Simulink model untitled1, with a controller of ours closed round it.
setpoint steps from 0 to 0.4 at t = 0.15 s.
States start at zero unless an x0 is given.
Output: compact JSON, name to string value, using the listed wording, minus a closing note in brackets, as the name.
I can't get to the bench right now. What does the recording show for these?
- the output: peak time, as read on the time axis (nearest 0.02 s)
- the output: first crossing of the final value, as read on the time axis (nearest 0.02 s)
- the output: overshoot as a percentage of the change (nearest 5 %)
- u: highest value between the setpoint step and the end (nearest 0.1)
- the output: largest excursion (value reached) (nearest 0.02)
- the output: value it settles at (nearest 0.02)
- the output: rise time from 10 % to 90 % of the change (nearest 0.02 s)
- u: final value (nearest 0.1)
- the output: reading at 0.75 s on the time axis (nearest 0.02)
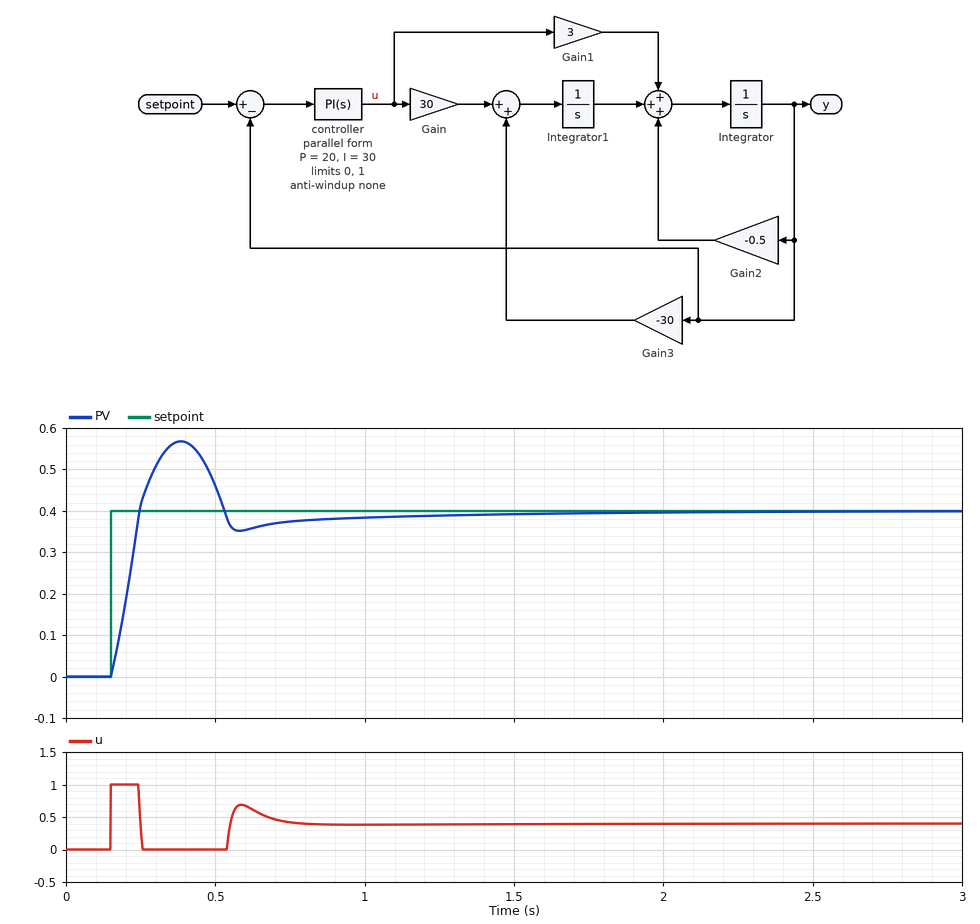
{"the output: peak time, as read on the time axis": "0.38 s", "the output: first crossing of the final value, as read on the time axis": "0.24 s", "the output: overshoot as a percentage of the change": "40 %", "u: highest value between the setpoint step and the end": "1.0", "the output: largest excursion (value reached)": "0.56", "the output: value it settles at": "0.40", "the output: rise time from 10 % to 90 % of the change": "0.08 s", "u: final value": "0.4", "the output: reading at 0.75 s on the time axis": "0.38"}
